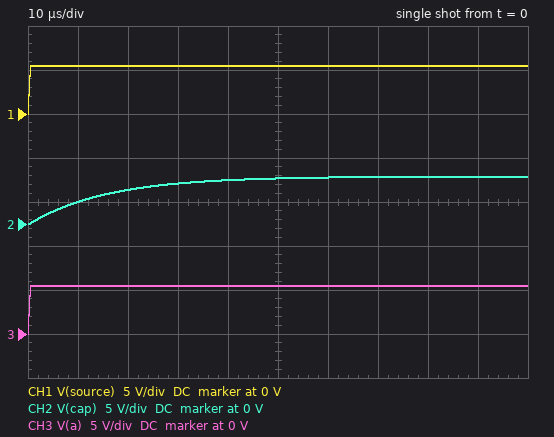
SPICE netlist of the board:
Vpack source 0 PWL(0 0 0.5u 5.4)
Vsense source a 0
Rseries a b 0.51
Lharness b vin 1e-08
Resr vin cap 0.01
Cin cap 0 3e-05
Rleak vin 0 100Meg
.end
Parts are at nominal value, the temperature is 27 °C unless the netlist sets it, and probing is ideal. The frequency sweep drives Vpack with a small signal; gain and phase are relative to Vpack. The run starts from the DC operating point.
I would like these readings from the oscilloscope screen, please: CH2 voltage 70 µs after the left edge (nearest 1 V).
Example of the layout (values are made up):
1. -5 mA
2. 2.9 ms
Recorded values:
1. 5 V
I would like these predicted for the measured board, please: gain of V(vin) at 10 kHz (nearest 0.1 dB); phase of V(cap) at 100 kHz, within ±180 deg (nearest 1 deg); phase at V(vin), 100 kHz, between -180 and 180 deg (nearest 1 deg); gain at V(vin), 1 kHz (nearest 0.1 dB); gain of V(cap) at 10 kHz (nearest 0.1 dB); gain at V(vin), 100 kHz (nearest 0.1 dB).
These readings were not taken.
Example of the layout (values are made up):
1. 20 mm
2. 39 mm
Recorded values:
1. -2.9 dB
2. -85 deg
3. -74 deg
4. 0 dB
5. -2.9 dB
6. -19.7 dB
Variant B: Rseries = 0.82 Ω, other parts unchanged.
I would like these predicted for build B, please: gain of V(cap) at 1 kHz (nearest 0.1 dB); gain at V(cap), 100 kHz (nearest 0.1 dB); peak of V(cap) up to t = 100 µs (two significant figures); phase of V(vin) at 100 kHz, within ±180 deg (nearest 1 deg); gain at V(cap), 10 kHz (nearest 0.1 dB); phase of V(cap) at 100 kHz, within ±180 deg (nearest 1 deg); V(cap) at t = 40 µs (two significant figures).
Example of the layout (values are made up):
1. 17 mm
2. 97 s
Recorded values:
1. -0.1 dB
2. -23.9 dB
3. 5.3 V
4. -76 deg
5. -5.4 dB
6. -87 deg
7. 4.3 V
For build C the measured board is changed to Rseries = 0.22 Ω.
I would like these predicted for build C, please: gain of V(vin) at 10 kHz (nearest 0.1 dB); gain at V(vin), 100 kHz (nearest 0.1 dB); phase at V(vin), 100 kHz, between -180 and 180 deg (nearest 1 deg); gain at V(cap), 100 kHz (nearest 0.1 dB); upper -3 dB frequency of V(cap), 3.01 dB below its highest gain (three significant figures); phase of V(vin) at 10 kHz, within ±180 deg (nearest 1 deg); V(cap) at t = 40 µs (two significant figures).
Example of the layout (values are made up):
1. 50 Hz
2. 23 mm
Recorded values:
1. -0.7 dB
2. -12.8 dB
3. -68 deg
4. -12.9 dB
5. 23.2 kHz
6. -22 deg
7. 5.4 V
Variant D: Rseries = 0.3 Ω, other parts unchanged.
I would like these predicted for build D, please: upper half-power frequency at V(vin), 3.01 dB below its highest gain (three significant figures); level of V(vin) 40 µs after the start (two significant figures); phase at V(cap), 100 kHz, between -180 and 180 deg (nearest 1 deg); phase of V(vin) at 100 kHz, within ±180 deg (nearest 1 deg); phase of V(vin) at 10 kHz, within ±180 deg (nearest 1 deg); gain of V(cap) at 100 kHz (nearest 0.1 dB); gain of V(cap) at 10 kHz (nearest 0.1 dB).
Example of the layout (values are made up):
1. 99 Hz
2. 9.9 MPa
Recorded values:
1. 17.2 kHz
2. 5.3 V
3. -81 deg
4. -71 deg
5. -29 deg
6. -15.4 dB
7. -1.3 dB
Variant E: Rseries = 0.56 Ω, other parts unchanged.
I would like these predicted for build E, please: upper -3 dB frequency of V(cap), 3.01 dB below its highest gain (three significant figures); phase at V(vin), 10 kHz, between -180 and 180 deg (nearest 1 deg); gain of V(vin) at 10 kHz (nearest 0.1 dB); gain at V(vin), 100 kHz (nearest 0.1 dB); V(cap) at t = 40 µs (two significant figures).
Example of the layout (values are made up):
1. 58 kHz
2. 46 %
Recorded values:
1. 9.32 kHz
2. -46 deg
3. -3.3 dB
4. -20.5 dB
5. 4.9 V
